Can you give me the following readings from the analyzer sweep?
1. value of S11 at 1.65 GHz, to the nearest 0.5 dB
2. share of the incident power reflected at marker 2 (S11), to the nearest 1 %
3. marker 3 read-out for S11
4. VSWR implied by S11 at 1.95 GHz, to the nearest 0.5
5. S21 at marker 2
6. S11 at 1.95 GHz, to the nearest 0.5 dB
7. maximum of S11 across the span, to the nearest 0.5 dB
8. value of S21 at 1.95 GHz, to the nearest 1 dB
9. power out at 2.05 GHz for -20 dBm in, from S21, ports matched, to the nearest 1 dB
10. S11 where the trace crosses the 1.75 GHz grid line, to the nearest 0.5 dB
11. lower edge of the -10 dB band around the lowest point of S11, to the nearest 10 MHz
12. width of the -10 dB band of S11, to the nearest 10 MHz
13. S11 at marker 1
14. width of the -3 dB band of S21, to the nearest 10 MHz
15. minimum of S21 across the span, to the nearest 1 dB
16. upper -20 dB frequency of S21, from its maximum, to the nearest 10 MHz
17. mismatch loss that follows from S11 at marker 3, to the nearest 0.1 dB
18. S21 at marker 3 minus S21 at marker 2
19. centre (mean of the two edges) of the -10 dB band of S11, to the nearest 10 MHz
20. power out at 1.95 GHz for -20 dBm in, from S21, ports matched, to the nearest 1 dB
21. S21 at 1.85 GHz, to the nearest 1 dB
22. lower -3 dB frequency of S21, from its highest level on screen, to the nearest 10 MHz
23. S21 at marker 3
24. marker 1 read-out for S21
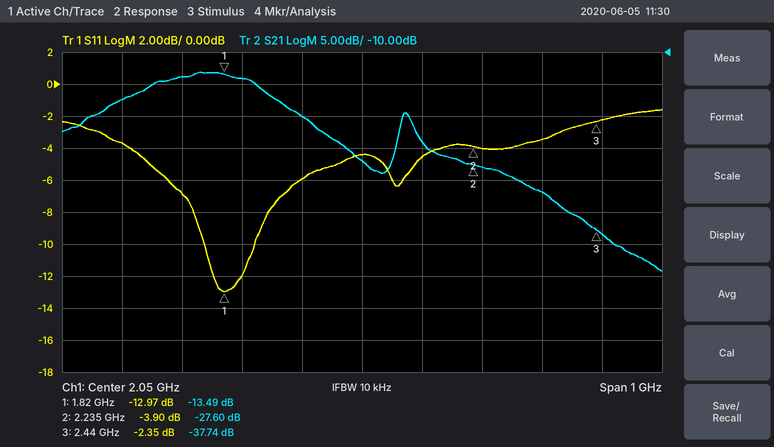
-3.5 dB
41 %
-2.35 dB
3.0
-27.60 dB
-6.0 dB
-1.5 dB
-20 dB
-47 dBm
-7.0 dB
1.79 GHz
80 MHz
-12.97 dB
210 MHz
-44 dB
2.37 GHz
3.8 dB
-10.14 dB
1.83 GHz
-40 dBm
-14 dB
1.68 GHz
-37.74 dB
-13.49 dB
